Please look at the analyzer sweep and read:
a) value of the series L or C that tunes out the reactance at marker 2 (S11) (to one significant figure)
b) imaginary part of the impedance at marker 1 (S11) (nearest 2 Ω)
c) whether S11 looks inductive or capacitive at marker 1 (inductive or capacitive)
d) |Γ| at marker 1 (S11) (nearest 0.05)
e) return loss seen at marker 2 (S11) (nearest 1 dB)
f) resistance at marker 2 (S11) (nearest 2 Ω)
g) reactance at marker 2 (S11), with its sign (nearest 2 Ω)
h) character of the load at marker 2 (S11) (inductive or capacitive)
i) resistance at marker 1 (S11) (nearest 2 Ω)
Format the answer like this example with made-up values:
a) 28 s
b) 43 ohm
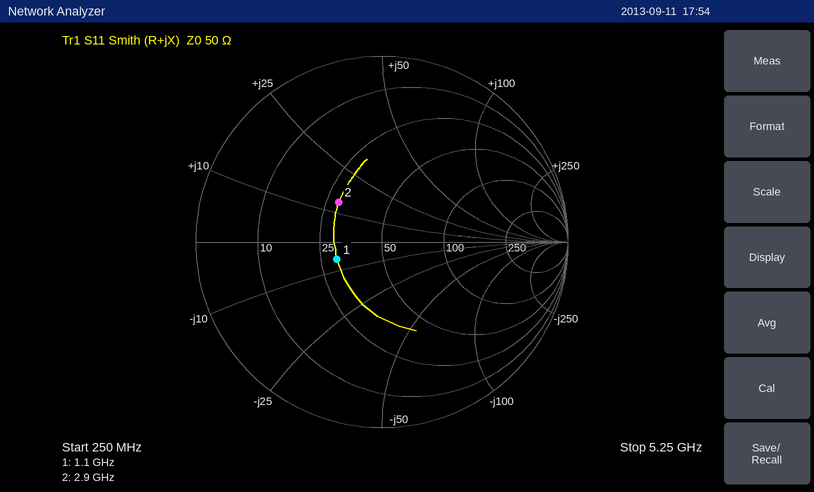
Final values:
a) 4 pF
b) -6 Ω
c) capacitive
d) 0.25
e) 10 dB
f) 28 Ω
g) +14 Ω
h) inductive
i) 30 Ω
